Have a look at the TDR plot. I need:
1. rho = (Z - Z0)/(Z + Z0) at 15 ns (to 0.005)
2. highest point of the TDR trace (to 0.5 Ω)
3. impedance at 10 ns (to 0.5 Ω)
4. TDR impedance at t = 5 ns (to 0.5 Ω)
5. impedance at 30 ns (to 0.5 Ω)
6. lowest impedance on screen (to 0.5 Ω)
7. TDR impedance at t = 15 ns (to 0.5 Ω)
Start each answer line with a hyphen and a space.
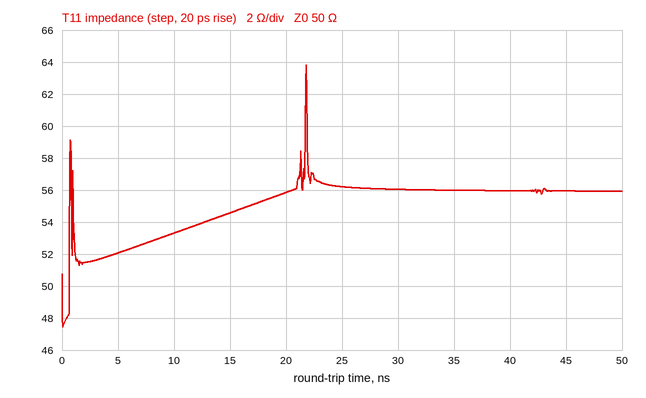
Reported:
- +0.045
- 64.0 Ω
- 53.5 Ω
- 52.0 Ω
- 56.0 Ω
- 47.5 Ω
- 54.5 Ω
